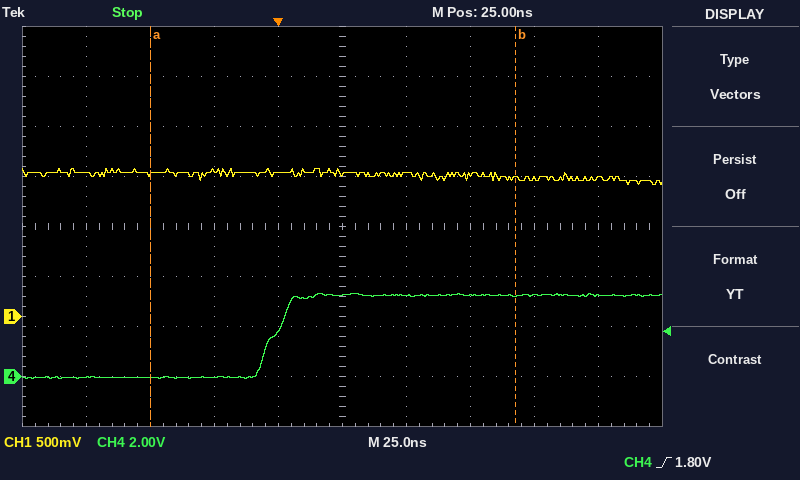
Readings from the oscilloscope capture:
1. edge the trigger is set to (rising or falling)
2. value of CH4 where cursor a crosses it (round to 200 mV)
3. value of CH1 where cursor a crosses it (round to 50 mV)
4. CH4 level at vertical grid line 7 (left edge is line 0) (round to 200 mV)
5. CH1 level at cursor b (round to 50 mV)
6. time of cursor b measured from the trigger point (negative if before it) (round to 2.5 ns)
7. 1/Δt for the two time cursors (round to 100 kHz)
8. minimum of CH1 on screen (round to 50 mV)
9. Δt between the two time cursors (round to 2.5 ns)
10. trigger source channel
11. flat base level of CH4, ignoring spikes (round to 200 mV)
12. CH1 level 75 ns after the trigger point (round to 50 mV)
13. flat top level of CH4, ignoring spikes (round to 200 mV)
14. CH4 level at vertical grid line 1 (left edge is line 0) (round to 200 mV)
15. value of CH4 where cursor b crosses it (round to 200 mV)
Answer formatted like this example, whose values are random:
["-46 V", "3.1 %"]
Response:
["rising", "0.0 V", "1.40 V", "3.2 V", "1.40 V", "+92.5 ns", "7.0 MHz", "1.30 V", "142.5 ns", "CH4", "0.0 V", "1.40 V", "3.2 V", "0.0 V", "3.2 V"]
